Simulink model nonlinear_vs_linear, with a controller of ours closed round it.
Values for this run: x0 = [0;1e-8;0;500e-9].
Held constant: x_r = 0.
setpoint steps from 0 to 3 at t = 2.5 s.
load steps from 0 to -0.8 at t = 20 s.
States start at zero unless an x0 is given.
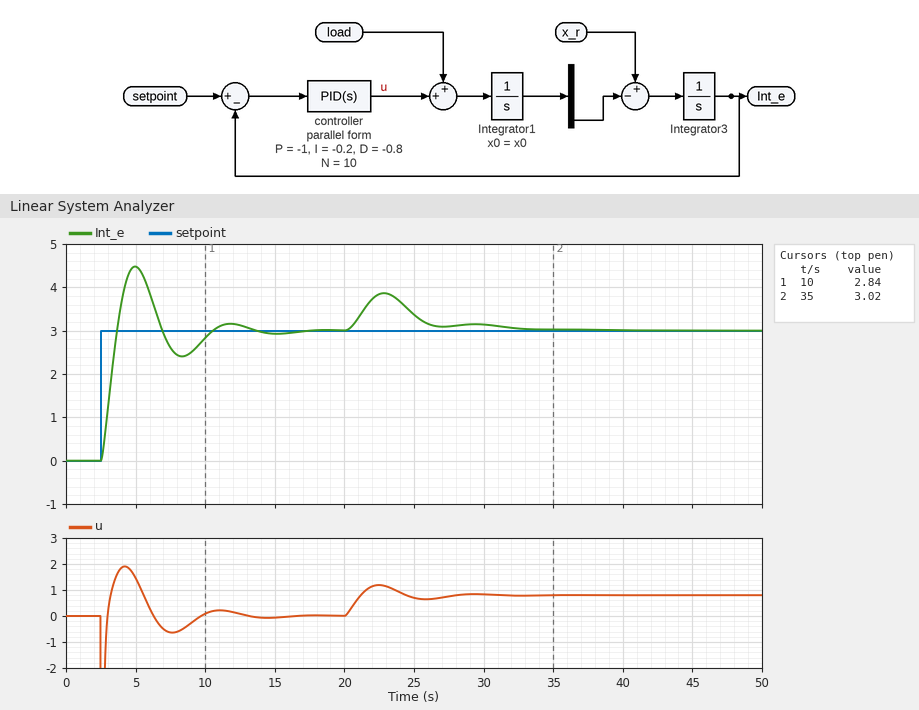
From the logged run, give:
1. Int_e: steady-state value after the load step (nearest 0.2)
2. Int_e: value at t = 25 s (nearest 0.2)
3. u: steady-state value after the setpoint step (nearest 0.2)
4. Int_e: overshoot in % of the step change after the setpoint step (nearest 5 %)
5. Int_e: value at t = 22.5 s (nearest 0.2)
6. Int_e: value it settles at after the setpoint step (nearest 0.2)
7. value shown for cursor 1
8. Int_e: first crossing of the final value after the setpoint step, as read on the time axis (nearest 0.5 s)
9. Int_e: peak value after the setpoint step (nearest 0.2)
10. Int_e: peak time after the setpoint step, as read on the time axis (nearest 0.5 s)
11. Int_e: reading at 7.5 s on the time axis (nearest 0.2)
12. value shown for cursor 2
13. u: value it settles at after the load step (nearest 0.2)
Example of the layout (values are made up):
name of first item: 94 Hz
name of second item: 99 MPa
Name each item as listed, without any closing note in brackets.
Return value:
Int_e: steady-state value after the load step: 3.0
Int_e: value at t = 25 s: 3.4
u: steady-state value after the setpoint step: 0.0
Int_e: overshoot in % of the step change after the setpoint step: 50 %
Int_e: value at t = 22.5 s: 3.8
Int_e: value it settles at after the setpoint step: 3.0
value shown for cursor 1: 2.84
Int_e: first crossing of the final value after the setpoint step, as read on the time axis: 3.5 s
Int_e: peak value after the setpoint step: 4.4
Int_e: peak time after the setpoint step, as read on the time axis: 5.0 s
Int_e: reading at 7.5 s on the time axis: 2.6
value shown for cursor 2: 3.02
u: value it settles at after the load step: 0.8
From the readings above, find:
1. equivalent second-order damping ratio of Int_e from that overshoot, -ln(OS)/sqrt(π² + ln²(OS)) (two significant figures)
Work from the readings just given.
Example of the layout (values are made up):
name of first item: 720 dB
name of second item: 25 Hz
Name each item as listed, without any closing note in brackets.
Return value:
equivalent second-order damping ratio of Int_e from that overshoot, -ln(OS)/sqrt(π² + ln²(OS)): 0.22
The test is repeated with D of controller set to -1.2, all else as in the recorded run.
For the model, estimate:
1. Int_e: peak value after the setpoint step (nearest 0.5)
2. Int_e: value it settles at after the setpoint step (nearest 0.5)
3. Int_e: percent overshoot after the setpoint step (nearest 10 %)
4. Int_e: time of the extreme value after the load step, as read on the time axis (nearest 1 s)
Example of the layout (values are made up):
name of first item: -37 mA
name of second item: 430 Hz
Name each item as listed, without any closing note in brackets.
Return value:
Int_e: peak value after the setpoint step: 4.0
Int_e: value it settles at after the setpoint step: 3.0
Int_e: percent overshoot after the setpoint step: 30 %
Int_e: time of the extreme value after the load step, as read on the time axis: 23 s
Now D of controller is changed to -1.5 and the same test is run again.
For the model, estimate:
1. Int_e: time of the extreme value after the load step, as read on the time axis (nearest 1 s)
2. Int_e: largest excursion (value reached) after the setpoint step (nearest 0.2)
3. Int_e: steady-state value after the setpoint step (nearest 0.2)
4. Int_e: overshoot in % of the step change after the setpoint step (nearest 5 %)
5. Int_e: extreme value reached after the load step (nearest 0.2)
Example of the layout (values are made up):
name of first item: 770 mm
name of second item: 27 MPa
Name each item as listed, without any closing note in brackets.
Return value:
Int_e: time of the extreme value after the load step, as read on the time axis: 23 s
Int_e: largest excursion (value reached) after the setpoint step: 3.8
Int_e: steady-state value after the setpoint step: 3.0
Int_e: overshoot in % of the step change after the setpoint step: 25 %
Int_e: extreme value reached after the load step: 3.6
